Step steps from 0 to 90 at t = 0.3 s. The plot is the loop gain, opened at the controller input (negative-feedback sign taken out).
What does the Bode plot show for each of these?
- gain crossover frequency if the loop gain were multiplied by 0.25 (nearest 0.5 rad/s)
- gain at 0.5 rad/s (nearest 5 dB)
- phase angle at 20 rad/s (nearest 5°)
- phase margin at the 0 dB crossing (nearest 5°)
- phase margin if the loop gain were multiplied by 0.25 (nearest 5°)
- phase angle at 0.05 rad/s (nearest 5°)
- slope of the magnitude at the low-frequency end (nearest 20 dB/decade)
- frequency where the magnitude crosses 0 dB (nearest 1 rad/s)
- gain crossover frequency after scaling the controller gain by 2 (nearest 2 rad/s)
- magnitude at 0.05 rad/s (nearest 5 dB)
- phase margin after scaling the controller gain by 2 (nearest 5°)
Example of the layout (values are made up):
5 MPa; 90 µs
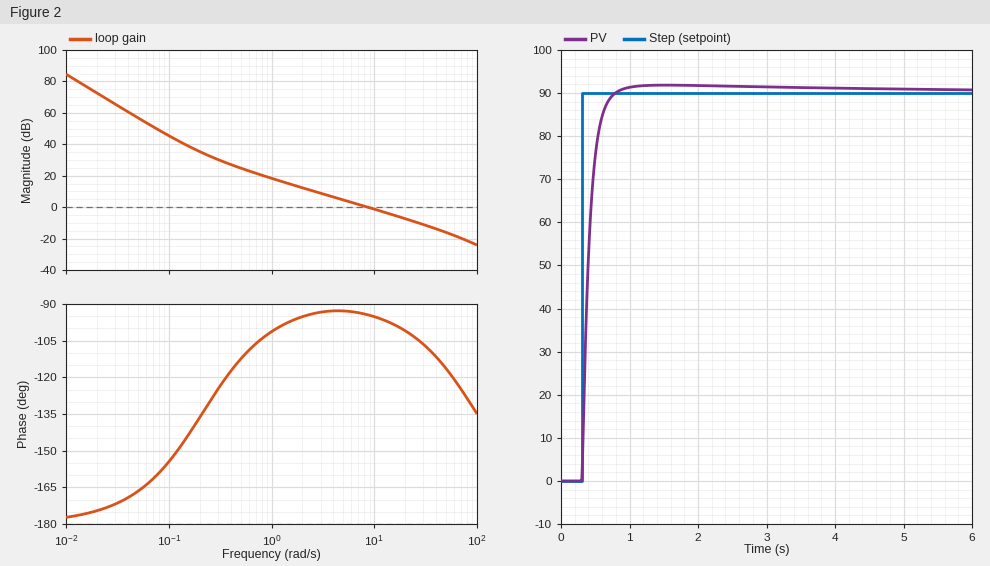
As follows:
2.0 rad/s; 25 dB; -100°; 85°; 85°; -165°; -40 dB/decade; 9 rad/s; 18 rad/s; 55 dB; 80°
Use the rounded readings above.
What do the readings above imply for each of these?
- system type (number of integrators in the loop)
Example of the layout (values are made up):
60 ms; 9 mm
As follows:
2
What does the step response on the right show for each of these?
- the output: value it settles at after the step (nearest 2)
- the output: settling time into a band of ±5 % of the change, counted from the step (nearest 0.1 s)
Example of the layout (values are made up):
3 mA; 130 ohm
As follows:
90; 0.3 s
